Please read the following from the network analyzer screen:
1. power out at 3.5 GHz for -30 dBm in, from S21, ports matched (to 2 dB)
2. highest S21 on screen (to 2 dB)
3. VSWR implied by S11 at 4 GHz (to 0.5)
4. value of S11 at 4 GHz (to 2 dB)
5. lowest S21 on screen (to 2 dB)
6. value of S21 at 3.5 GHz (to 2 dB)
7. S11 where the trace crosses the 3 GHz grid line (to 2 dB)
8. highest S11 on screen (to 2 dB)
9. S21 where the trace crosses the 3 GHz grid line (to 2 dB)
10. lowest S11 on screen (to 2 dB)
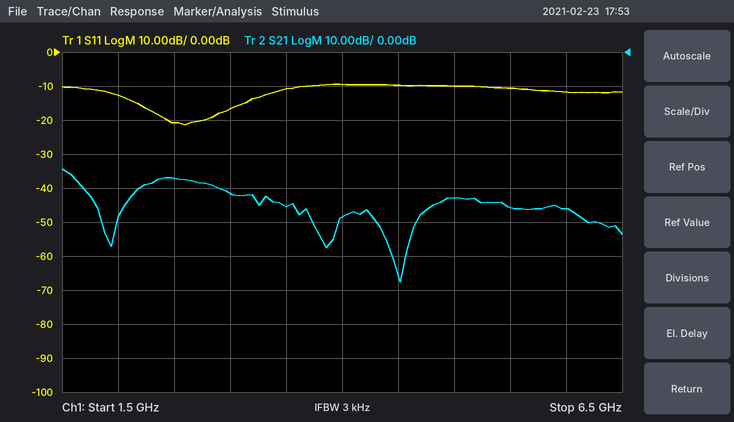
-76 dBm
-34 dB
2.0
-10 dB
-68 dB
-46 dB
-16 dB
-10 dB
-42 dB
-22 dB
